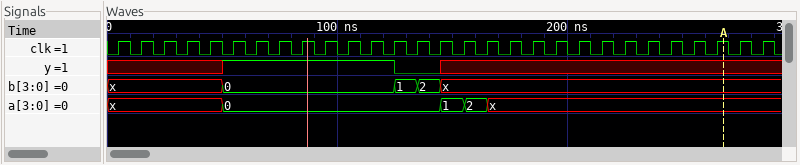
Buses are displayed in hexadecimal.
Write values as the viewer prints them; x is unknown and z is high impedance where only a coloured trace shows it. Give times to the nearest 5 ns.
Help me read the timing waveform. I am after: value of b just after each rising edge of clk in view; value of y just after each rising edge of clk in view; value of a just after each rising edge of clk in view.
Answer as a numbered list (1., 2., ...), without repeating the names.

1. x, x, x, x, x, 0, 0, 0, 0, 0, 0, 0, 1, 2, x, x, x, x, x, x, x, x, x, x, x, x, x, x, x
2. x x x x x 1 1 1 1 1 1 1 0 0 x x x x x x x x x x x x x x x
3. x, x, x, x, x, 0, 0, 0, 0, 0, 0, 0, 0, 0, 1, 2, x, x, x, x, x, x, x, x, x, x, x, x, x
